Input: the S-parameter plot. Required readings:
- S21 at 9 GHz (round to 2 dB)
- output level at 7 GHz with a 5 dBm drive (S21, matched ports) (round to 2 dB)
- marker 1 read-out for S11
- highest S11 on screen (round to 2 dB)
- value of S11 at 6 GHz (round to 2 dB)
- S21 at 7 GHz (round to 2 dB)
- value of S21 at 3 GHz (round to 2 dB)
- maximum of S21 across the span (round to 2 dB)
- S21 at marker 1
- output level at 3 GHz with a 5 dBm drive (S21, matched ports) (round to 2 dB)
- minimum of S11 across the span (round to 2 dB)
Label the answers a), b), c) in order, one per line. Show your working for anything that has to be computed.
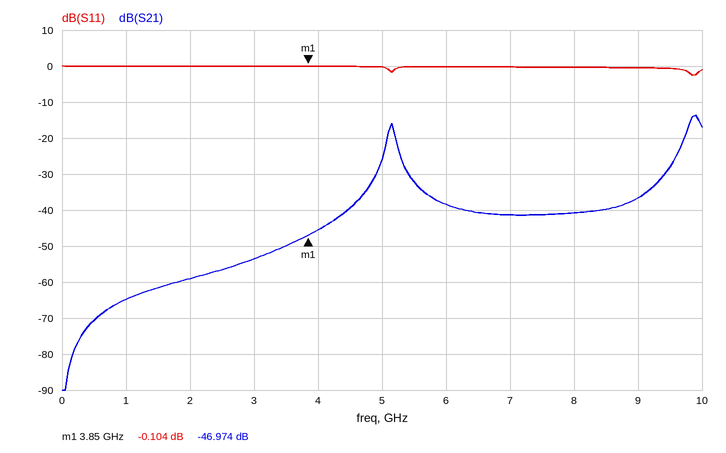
a) -36 dB
b) 5 dBm + (-42 dB) = -36 dBm
c) -0.104 dB
d) 0 dB
e) 0 dB
f) -42 dB
g) -54 dB
h) -14 dB
i) -46.974 dB
j) 5 dBm + (-54 dB) = -48 dBm
k) -2 dB
